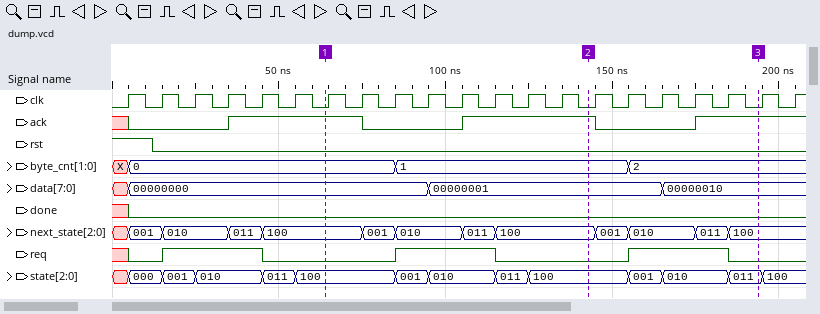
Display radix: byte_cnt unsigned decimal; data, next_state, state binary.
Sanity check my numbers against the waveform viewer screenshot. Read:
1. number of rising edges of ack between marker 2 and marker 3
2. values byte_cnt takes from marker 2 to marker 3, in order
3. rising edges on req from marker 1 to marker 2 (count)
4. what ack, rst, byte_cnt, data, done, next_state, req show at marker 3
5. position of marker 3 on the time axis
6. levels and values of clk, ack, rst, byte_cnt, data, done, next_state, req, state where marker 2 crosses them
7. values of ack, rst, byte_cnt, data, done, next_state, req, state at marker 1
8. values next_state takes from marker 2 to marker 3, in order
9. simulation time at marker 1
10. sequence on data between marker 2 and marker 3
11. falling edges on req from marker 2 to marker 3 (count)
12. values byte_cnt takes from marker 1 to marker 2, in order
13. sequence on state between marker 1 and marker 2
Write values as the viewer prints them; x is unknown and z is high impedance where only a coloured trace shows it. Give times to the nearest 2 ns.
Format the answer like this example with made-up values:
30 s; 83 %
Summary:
1; 1, 2; 1; ack=1, rst=0, byte_cnt=2, data=00000010, done=0, next_state=100, req=0; 194 ns; clk=0, ack=1, rst=0, byte_cnt=1, data=00000001, done=0, next_state=100, req=0, state=100; ack=1, rst=0, byte_cnt=0, data=00000000, done=0, next_state=100, req=0, state=100; 100, 001, 010, 011, 100; 64 ns; 00000001, 00000010; 1; 0, 1; 100, 001, 010, 011, 100
